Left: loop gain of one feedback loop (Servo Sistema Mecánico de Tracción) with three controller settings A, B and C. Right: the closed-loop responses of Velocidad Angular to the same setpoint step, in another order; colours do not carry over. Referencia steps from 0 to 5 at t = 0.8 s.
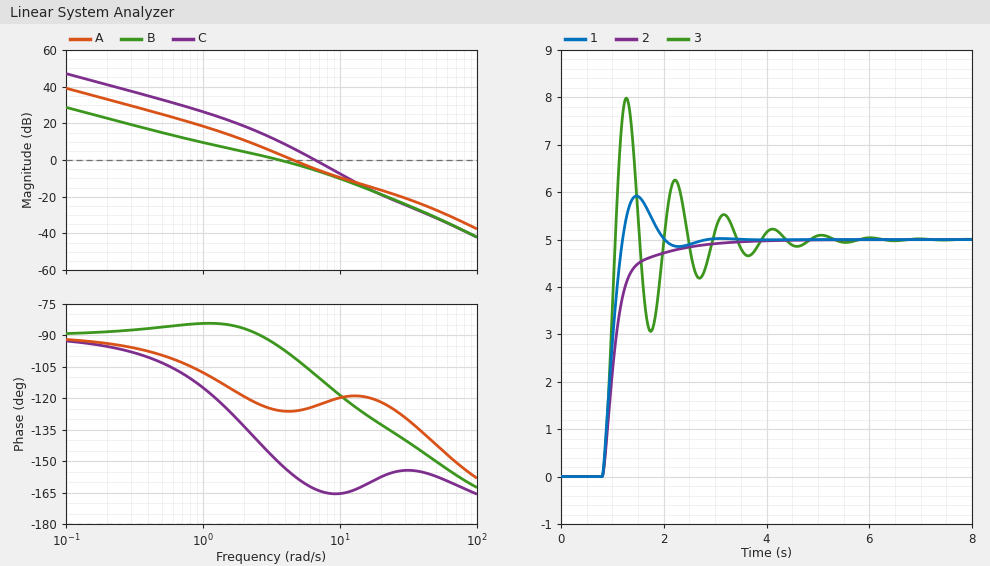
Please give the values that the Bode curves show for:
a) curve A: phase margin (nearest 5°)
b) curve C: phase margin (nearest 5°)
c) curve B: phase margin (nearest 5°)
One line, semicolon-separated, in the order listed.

55°; 15°; 85°
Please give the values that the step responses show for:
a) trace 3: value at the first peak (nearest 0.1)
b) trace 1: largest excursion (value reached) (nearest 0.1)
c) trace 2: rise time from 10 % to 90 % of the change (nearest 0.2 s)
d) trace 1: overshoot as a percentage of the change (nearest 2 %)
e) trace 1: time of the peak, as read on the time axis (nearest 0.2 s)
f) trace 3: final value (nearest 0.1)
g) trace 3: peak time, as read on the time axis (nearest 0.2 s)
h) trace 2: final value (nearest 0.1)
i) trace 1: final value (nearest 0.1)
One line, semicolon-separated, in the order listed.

8.0; 5.9; 0.6 s; 18 %; 1.4 s; 5.0; 1.2 s; 5.0; 5.0
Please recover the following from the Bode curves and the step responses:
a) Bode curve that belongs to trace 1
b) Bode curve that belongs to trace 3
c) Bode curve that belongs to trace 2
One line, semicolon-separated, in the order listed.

A; C; B
